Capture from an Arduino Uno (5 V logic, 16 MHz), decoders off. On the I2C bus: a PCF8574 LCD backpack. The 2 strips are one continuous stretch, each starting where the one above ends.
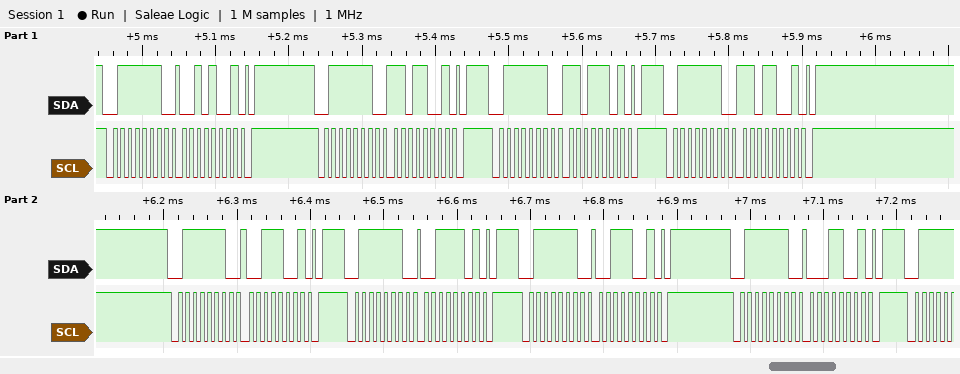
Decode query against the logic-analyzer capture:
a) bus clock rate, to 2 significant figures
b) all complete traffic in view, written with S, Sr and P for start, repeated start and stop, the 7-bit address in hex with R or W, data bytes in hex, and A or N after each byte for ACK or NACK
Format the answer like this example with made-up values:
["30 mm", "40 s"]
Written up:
["100 kHz", "S 3FW A 29 A P S 3FW A D9 A P S 3FW A DD A P S 3FW A D9 A P S 3FW A 39 A P S 3FW A 3D A P S 3FW A 39 A P S 3FW A 19 A P"]
